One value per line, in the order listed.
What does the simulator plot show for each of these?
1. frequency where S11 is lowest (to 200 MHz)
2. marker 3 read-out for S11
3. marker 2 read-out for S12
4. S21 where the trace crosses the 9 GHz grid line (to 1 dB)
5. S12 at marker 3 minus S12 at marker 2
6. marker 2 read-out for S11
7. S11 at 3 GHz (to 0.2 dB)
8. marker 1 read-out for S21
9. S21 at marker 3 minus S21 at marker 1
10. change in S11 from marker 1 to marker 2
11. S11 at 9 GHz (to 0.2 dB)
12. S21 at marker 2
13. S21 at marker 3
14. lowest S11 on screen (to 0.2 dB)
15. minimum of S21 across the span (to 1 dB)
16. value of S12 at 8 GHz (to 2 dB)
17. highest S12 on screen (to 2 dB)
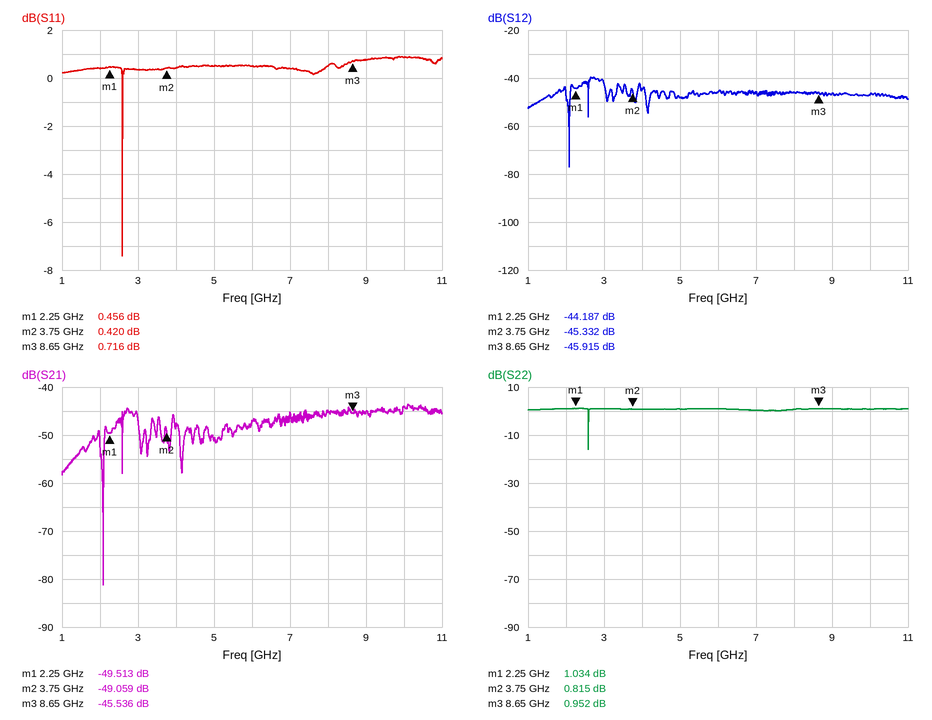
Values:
2.6 GHz
0.716 dB
-45.332 dB
-45 dB
-0.583 dB
0.420 dB
0.4 dB
-49.513 dB
3.977 dB
-0.036 dB
0.8 dB
-49.059 dB
-45.536 dB
-7.4 dB
-81 dB
-46 dB
-40 dB
